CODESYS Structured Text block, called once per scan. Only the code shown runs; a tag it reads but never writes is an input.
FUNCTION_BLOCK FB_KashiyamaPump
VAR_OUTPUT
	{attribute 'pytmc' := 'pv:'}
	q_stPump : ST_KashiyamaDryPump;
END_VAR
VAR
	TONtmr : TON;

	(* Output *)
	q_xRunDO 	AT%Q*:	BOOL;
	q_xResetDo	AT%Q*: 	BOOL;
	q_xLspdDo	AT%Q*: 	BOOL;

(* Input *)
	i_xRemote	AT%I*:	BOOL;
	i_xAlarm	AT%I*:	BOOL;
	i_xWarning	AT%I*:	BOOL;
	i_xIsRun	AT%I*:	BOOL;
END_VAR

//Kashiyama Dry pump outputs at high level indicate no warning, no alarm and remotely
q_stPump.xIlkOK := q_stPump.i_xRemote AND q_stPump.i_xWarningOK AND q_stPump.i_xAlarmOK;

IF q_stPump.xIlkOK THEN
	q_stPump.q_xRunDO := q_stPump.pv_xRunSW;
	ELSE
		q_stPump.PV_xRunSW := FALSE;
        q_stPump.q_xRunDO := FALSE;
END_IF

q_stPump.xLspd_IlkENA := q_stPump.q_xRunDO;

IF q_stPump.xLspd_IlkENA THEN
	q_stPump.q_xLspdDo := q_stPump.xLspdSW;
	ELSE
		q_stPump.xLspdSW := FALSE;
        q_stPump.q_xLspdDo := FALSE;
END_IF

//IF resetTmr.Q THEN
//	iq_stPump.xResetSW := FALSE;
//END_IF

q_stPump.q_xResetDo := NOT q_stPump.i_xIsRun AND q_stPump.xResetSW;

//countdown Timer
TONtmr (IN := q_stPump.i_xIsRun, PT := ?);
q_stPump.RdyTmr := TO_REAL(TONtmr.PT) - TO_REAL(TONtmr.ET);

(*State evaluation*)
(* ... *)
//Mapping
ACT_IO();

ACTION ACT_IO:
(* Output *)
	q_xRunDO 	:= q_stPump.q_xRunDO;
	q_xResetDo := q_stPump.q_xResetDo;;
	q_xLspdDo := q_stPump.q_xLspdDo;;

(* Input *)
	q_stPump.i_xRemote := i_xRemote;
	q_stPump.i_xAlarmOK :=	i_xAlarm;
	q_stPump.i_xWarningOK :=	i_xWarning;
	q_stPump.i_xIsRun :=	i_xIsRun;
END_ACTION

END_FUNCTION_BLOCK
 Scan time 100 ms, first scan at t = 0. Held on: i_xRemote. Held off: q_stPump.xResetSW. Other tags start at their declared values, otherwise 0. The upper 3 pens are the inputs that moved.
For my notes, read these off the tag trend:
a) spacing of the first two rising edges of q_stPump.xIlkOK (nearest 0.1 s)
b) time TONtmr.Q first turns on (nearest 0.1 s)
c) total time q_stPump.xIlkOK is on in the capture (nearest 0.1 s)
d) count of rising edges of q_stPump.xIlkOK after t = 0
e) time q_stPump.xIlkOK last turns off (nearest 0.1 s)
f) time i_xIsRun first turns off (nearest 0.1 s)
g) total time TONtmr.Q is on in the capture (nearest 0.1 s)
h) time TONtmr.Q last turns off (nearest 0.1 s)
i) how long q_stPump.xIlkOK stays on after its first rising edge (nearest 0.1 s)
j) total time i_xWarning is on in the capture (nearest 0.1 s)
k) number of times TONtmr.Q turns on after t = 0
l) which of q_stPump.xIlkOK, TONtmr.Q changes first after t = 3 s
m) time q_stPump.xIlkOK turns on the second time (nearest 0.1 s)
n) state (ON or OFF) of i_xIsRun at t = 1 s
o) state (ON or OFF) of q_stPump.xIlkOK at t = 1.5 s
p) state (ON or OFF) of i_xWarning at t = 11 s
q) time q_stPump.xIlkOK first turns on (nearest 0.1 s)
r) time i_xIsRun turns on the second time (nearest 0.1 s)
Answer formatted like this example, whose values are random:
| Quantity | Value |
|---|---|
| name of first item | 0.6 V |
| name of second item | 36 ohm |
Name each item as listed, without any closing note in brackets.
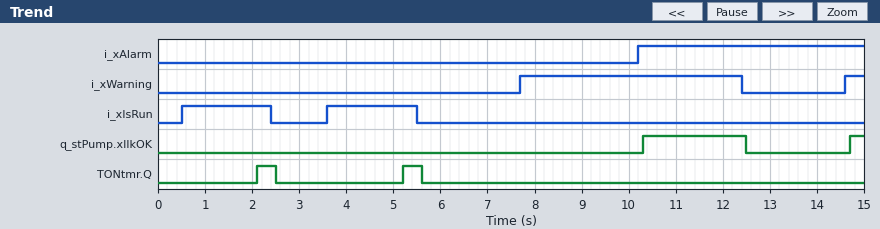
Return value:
| Quantity | Value |
|---|---|
| spacing of the first two rising edges of q_stPump.xIlkOK | 4.4 s |
| time TONtmr.Q first turns on | 2.1 s |
| total time q_stPump.xIlkOK is on in the capture | 2.5 s |
| count of rising edges of q_stPump.xIlkOK after t = 0 | 2 |
| time q_stPump.xIlkOK last turns off | 12.5 s |
| time i_xIsRun first turns off | 2.4 s |
| total time TONtmr.Q is on in the capture | 0.8 s |
| time TONtmr.Q last turns off | 5.6 s |
| how long q_stPump.xIlkOK stays on after its first rising edge | 2.2 s |
| total time i_xWarning is on in the capture | 5.1 s |
| number of times TONtmr.Q turns on after t = 0 | 2 |
| which of q_stPump.xIlkOK, TONtmr.Q changes first after t = 3 s | TONtmr.Q |
| time q_stPump.xIlkOK turns on the second time | 14.7 s |
| state (ON or OFF) of i_xIsRun at t = 1 s | ON |
| state (ON or OFF) of q_stPump.xIlkOK at t = 1.5 s | OFF |
| state (ON or OFF) of i_xWarning at t = 11 s | ON |
| time q_stPump.xIlkOK first turns on | 10.3 s |
| time i_xIsRun turns on the second time | 3.6 s |
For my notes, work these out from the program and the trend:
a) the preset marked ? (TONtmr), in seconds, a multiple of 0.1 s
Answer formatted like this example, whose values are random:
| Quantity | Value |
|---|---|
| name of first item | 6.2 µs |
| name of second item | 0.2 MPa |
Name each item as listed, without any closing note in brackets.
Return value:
| Quantity | Value |
|---|---|
| the preset marked ? (TONtmr), in seconds, a multiple of 0.1 s | 1.5 s |
